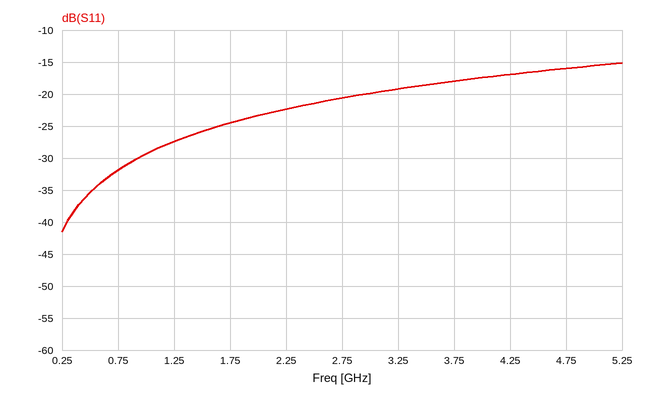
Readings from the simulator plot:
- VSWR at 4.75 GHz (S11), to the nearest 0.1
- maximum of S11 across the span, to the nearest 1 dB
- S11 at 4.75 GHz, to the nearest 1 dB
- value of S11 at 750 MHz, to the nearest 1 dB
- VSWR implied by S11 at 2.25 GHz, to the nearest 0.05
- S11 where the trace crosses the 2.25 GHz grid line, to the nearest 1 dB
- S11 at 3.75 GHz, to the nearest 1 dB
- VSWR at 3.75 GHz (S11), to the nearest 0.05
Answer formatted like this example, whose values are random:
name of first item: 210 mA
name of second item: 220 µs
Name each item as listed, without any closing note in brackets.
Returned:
VSWR at 4.75 GHz (S11), to the nearest 0.1: 1.4
maximum of S11 across the span, to the nearest 1 dB: -15 dB
S11 at 4.75 GHz, to the nearest 1 dB: -16 dB
value of S11 at 750 MHz, to the nearest 1 dB: -32 dB
VSWR implied by S11 at 2.25 GHz, to the nearest 0.05: 1.15
S11 where the trace crosses the 2.25 GHz grid line, to the nearest 1 dB: -22 dB
S11 at 3.75 GHz, to the nearest 1 dB: -18 dB
VSWR at 3.75 GHz (S11), to the nearest 0.05: 1.30
